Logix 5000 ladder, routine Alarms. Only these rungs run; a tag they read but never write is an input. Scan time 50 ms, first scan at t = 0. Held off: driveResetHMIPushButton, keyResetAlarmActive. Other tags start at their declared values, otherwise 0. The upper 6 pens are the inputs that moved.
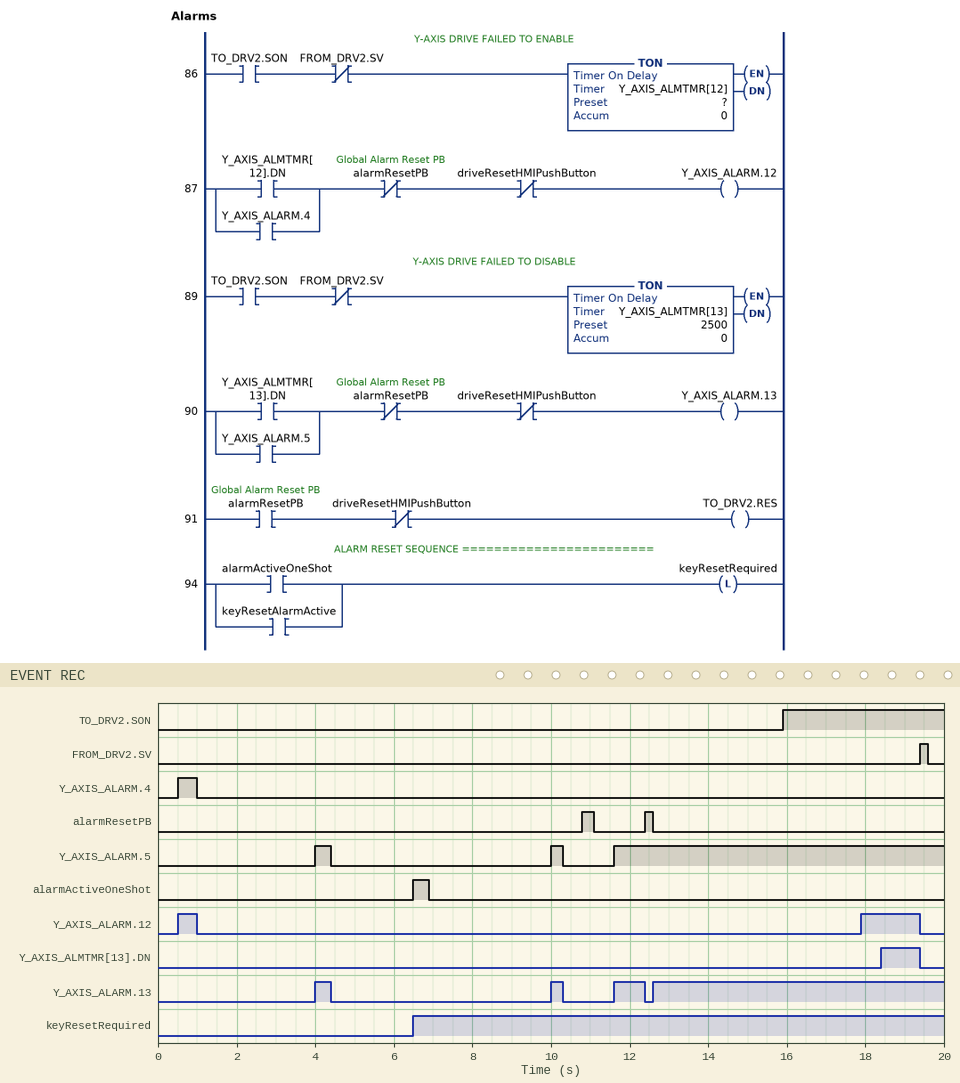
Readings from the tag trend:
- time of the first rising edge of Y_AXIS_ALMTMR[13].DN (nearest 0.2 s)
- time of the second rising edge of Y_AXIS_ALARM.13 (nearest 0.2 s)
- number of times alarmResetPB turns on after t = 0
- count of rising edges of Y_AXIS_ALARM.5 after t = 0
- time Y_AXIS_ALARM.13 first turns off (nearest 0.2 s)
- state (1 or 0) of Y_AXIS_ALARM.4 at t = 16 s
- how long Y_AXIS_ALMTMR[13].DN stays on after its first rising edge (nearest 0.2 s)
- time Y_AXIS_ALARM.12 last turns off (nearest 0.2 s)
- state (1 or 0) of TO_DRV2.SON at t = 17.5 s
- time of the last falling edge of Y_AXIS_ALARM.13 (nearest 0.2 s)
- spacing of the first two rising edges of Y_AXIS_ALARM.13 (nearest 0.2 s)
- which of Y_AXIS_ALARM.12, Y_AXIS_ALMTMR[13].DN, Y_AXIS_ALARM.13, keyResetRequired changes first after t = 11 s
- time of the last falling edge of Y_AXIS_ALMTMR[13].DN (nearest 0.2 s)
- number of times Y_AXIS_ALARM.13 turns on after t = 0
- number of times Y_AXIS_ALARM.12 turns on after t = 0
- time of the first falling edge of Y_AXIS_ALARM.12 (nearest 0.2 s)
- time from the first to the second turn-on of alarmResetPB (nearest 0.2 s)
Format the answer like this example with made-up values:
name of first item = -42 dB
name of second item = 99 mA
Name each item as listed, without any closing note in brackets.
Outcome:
time of the first rising edge of Y_AXIS_ALMTMR[13].DN = 18.4 s
time of the second rising edge of Y_AXIS_ALARM.13 = 10.0 s
number of times alarmResetPB turns on after t = 0 = 2
count of rising edges of Y_AXIS_ALARM.5 after t = 0 = 3
time Y_AXIS_ALARM.13 first turns off = 4.4 s
state (1 or 0) of Y_AXIS_ALARM.4 at t = 16 s = 0
how long Y_AXIS_ALMTMR[13].DN stays on after its first rising edge = 1.0 s
time Y_AXIS_ALARM.12 last turns off = 19.4 s
state (1 or 0) of TO_DRV2.SON at t = 17.5 s = 1
time of the last falling edge of Y_AXIS_ALARM.13 = 12.4 s
spacing of the first two rising edges of Y_AXIS_ALARM.13 = 6.0 s
which of Y_AXIS_ALARM.12, Y_AXIS_ALMTMR[13].DN, Y_AXIS_ALARM.13, keyResetRequired changes first after t = 11 s = Y_AXIS_ALARM.13
time of the last falling edge of Y_AXIS_ALMTMR[13].DN = 19.4 s
number of times Y_AXIS_ALARM.13 turns on after t = 0 = 4
number of times Y_AXIS_ALARM.12 turns on after t = 0 = 2
time of the first falling edge of Y_AXIS_ALARM.12 = 1.0 s
time from the first to the second turn-on of alarmResetPB = 1.6 s
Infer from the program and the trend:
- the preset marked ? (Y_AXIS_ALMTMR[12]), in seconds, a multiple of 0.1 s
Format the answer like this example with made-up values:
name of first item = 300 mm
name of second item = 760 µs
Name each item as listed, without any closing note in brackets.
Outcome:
the preset marked ? (Y_AXIS_ALMTMR[12]), in seconds, a multiple of 0.1 s = 2.0 s
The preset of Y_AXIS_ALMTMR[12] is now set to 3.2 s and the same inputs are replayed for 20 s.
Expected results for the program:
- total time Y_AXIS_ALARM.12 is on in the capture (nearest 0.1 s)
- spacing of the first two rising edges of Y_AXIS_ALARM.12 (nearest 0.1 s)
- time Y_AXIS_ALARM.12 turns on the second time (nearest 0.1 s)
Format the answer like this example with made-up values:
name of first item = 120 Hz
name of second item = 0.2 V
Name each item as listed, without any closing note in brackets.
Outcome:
total time Y_AXIS_ALARM.12 is on in the capture = 0.8 s
spacing of the first two rising edges of Y_AXIS_ALARM.12 = 18.6 s
time Y_AXIS_ALARM.12 turns on the second time = 19.1 s
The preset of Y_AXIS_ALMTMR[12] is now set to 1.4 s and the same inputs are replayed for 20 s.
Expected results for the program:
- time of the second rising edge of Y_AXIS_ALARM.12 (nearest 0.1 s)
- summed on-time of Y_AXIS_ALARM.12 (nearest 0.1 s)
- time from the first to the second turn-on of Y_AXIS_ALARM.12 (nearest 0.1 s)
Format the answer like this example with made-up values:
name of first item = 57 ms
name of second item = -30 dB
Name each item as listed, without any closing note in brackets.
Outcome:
time of the second rising edge of Y_AXIS_ALARM.12 = 17.3 s
summed on-time of Y_AXIS_ALARM.12 = 2.6 s
time from the first to the second turn-on of Y_AXIS_ALARM.12 = 16.8 s
